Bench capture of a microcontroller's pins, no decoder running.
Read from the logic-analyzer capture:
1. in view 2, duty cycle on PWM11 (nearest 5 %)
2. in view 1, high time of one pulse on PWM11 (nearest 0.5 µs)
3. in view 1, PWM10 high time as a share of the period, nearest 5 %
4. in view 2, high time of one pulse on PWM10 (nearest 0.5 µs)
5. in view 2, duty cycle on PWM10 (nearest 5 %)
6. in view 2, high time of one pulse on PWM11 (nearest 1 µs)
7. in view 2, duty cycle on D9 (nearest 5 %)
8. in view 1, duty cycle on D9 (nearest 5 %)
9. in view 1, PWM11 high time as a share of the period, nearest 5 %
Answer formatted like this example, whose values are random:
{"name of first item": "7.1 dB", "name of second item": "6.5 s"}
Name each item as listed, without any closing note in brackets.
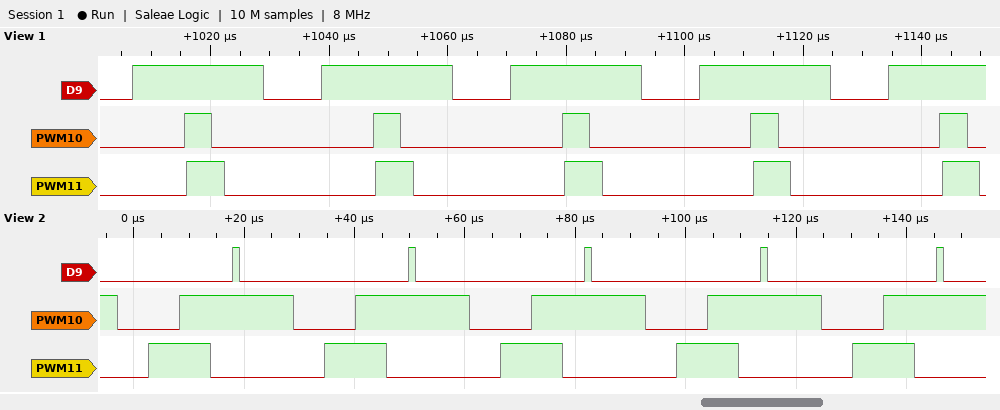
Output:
{"in view 2, duty cycle on PWM11": "35 %", "in view 1, high time of one pulse on PWM11": "6.5 µs", "in view 1, PWM10 high time as a share of the period, nearest 5 %": "15 %", "in view 2, high time of one pulse on PWM10": "20.5 µs", "in view 2, duty cycle on PWM10": "65 %", "in view 2, high time of one pulse on PWM11": "11 µs", "in view 2, duty cycle on D9": "5 %", "in view 1, duty cycle on D9": "70 %", "in view 1, PWM11 high time as a share of the period, nearest 5 %": "20 %"}
